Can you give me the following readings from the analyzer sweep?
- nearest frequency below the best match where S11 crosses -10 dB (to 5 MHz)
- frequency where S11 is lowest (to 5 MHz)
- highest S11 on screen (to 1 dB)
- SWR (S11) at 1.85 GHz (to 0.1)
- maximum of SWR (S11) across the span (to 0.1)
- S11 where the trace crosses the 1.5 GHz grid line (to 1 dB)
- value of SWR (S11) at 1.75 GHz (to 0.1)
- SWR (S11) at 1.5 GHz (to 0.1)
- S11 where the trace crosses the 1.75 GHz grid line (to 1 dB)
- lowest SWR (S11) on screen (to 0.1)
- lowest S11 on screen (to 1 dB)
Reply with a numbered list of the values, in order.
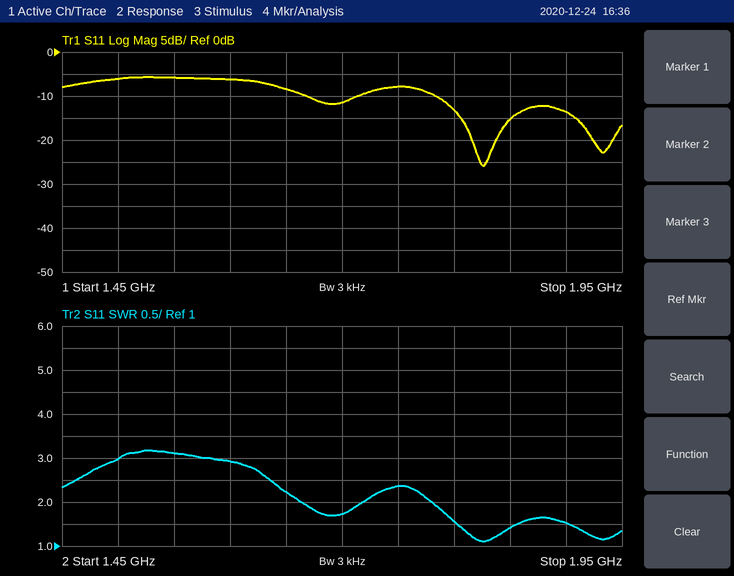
1. 1.785 GHz
2. 1.825 GHz
3. -6 dB
4. 1.4
5. 3.2
6. -6 dB
7. 2.4
8. 3.0
9. -8 dB
10. 1.1
11. -26 dB
